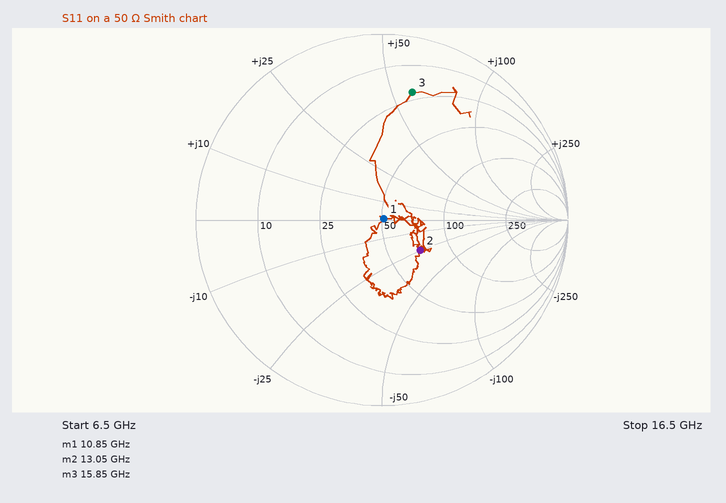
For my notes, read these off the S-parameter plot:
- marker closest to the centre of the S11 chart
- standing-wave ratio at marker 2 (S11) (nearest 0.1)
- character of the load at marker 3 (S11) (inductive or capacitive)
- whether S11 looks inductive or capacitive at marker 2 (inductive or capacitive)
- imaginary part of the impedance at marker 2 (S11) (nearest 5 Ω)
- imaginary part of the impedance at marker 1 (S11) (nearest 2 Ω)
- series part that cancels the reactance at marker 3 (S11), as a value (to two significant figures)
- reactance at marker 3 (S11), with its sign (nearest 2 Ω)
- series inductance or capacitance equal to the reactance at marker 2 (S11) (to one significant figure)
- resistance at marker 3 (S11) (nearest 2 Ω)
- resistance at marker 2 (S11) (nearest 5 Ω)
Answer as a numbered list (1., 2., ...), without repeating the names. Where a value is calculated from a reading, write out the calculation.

1. marker 1
2. 1.7
3. inductive
4. capacitive
5. -25 Ω
6. 0 Ω
7. C = 1/(2π × 15.85 GHz × 58 Ω) ≈ 173 fF, so 170 fF to two significant figures
8. +58 Ω
9. C = 1/(2π × 13.05 GHz × 25 Ω) ≈ 488 fF, so 500 fF to one significant figure
10. 22 Ω
11. 70 Ω
